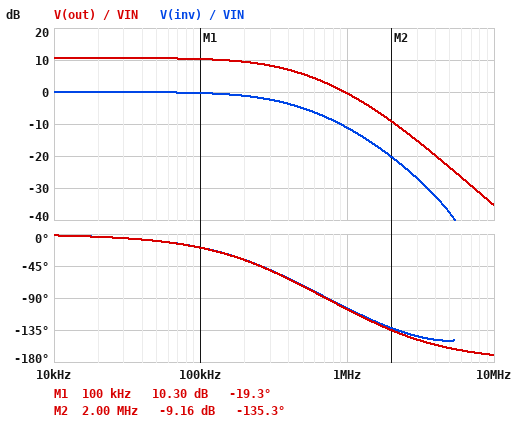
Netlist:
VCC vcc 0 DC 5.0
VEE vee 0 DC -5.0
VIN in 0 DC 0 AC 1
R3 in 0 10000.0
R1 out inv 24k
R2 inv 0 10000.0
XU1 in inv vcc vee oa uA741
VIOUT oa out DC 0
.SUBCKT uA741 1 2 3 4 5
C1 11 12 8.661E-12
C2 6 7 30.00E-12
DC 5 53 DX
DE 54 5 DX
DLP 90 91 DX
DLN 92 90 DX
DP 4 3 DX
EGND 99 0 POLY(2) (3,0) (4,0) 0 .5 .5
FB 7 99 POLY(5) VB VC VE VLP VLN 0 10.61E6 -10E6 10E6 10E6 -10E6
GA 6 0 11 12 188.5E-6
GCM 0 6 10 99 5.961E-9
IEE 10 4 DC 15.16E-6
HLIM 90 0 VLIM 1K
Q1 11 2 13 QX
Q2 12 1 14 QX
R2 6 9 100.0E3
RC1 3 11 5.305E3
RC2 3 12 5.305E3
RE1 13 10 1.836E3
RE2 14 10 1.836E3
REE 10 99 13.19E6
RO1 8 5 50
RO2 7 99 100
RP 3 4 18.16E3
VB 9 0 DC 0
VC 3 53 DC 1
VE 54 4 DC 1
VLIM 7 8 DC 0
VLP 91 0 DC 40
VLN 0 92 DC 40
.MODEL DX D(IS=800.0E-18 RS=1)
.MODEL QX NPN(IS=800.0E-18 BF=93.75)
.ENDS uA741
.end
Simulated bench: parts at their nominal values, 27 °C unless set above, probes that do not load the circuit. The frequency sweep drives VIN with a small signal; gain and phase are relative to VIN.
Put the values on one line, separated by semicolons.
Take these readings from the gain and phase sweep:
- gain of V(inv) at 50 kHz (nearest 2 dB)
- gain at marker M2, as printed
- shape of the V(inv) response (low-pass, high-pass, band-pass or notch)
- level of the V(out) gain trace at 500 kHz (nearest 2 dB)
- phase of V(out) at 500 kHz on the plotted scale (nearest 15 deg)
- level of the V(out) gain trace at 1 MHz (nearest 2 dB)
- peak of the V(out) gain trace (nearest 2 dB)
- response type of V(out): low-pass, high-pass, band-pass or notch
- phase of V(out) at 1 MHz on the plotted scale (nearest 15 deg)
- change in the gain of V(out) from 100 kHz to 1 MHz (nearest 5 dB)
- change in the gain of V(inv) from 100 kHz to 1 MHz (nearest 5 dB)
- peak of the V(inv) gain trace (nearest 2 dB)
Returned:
0 dB; -9.16 dB; low-pass; 6 dB; -75 deg; 0 dB; 10 dB; low-pass; -105 deg; -10 dB; -10 dB; 0 dB
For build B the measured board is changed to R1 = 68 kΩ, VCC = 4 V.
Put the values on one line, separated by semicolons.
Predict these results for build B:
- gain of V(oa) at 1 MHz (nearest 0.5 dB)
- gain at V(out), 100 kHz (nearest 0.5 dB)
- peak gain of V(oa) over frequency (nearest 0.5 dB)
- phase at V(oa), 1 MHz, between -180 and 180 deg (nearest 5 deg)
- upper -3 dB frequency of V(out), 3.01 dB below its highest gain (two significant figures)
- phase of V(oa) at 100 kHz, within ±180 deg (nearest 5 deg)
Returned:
-1.0 dB; 16.0 dB; 18.0 dB; -115 deg; 140 kHz; -40 deg
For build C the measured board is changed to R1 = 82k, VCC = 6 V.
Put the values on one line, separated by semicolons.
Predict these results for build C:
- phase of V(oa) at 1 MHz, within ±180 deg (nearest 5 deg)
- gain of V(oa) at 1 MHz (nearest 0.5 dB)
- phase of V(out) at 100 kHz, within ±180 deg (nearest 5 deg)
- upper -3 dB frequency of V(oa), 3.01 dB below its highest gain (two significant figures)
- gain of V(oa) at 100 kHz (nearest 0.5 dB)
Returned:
-115 deg; -1.0 dB; -45 deg; 110 kHz; 17.0 dB
